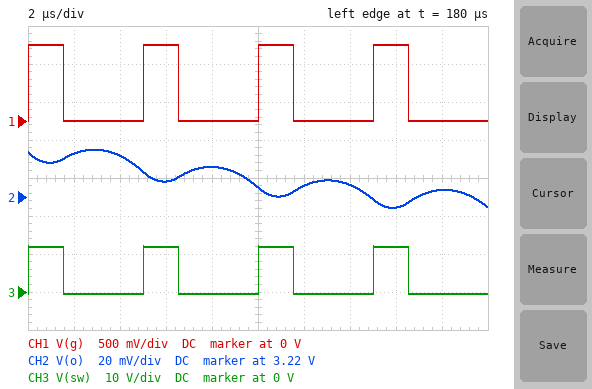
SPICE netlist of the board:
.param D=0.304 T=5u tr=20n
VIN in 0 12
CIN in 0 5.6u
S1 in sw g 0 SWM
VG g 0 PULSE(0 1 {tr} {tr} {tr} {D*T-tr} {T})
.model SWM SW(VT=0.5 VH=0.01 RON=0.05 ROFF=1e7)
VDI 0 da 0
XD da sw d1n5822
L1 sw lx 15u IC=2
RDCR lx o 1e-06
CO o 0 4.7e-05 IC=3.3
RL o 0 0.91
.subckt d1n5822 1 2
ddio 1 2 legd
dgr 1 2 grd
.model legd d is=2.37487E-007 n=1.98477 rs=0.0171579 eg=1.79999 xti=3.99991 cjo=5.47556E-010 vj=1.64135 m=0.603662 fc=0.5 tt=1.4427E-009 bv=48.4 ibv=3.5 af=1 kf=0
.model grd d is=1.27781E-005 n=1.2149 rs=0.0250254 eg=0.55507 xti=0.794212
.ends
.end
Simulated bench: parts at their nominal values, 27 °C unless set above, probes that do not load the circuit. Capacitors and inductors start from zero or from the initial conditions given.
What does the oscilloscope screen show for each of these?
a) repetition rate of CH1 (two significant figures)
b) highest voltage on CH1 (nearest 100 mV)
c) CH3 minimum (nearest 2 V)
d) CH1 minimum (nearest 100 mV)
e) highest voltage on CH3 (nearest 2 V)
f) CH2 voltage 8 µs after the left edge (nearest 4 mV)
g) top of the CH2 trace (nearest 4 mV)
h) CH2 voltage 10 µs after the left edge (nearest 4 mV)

200 kHz
1.0 V
0 V
0 V
12 V
3.236 V
3.244 V
3.224 V
